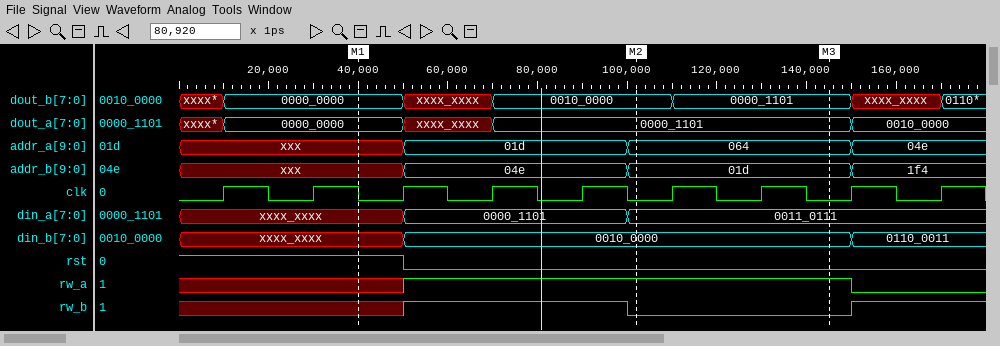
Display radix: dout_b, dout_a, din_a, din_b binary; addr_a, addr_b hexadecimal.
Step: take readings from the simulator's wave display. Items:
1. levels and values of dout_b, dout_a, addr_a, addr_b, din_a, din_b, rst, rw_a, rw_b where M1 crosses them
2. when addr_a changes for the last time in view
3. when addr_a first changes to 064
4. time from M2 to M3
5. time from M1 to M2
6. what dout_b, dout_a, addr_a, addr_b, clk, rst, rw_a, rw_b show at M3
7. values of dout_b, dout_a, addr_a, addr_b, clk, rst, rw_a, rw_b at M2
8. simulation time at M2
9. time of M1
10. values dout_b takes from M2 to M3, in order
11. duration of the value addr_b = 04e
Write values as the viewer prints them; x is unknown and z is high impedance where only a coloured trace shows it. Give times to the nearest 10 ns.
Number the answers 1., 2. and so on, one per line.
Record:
1. dout_b=0000_0000, dout_a=0000_0000, addr_a=xxx, addr_b=xxx, din_a=xxxx_xxxx, din_b=xxxx_xxxx, rst=1, rw_a=x, rw_b=x
2. 150 ns
3. 100 ns
4. 40 ns
5. 60 ns
6. dout_b=0000_1101, dout_a=0000_1101, addr_a=064, addr_b=01d, clk=0, rst=0, rw_a=1, rw_b=0
7. dout_b=0010_0000, dout_a=0000_1101, addr_a=064, addr_b=01d, clk=0, rst=0, rw_a=1, rw_b=0
8. 100 ns
9. 40 ns
10. 0010_0000, 0000_1101
11. 50 ns
